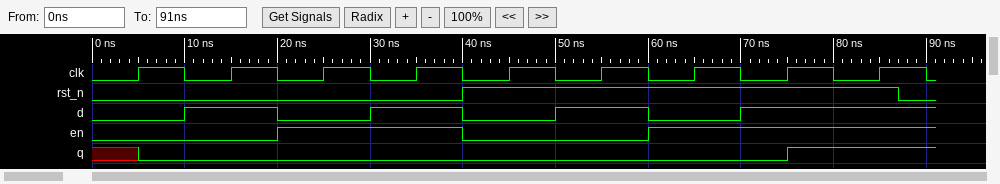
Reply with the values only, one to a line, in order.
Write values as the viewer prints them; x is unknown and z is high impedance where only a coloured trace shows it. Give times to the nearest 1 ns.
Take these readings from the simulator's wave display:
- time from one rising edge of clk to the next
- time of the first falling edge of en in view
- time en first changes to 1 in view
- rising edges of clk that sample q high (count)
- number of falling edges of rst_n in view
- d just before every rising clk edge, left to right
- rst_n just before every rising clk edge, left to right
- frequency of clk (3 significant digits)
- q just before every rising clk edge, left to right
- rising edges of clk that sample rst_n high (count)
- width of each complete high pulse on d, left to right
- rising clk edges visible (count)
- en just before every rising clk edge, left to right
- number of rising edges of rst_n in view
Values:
10 ns
40 ns
20 ns
1
1
0 1 0 1 0 1 0 1 1
0 0 0 0 1 1 1 1 1
100 MHz
x 0 0 0 0 0 0 0 1
5
10 ns, 10 ns, 10 ns
9
0 0 1 1 0 0 1 1 1
1
